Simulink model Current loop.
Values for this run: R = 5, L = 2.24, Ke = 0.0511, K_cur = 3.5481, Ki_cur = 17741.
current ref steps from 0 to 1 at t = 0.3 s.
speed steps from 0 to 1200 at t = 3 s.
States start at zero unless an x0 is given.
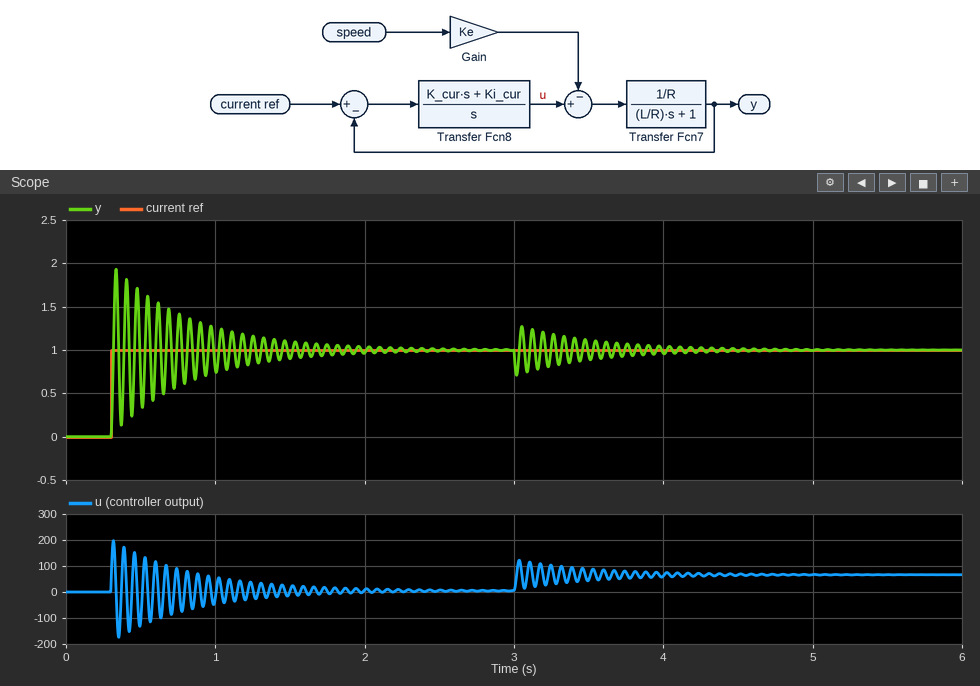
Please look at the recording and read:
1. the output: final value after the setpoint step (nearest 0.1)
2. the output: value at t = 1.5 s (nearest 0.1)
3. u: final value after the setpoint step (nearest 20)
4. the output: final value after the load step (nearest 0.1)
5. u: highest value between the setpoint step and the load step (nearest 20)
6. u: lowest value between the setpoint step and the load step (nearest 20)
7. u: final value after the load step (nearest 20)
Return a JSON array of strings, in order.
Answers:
["1.0", "0.9", "0", "1.0", "200", "-180", "60"]
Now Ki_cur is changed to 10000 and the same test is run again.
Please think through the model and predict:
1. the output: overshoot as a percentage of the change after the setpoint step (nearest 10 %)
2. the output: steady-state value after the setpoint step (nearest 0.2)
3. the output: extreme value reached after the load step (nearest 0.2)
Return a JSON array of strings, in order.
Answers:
["90 %", "1.0", "0.6"]
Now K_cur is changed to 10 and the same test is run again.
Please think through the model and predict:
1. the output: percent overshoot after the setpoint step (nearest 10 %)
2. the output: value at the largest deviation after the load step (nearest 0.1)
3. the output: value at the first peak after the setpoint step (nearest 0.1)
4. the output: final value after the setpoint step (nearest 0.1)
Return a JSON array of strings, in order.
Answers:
["90 %", "0.7", "1.9", "1.0"]
